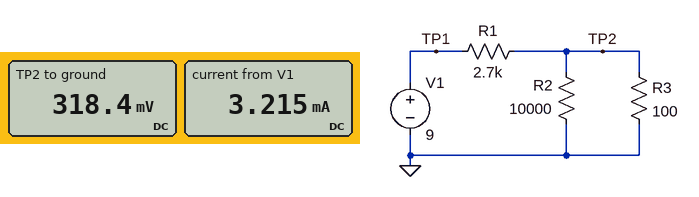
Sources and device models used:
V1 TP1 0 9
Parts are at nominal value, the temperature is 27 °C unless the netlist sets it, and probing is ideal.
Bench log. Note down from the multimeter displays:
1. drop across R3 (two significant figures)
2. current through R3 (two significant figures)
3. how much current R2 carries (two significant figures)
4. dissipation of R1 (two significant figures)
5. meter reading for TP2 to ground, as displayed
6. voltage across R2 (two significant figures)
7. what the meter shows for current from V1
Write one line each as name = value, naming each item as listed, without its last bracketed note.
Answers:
drop across R3 = 320 mV
current through R3 = 3.2 mA
how much current R2 carries = 32 µA
dissipation of R1 = 28 mW
meter reading for TP2 to ground, as displayed = 318.4 mV
voltage across R2 = 320 mV
what the meter shows for current from V1 = 3.215 mA
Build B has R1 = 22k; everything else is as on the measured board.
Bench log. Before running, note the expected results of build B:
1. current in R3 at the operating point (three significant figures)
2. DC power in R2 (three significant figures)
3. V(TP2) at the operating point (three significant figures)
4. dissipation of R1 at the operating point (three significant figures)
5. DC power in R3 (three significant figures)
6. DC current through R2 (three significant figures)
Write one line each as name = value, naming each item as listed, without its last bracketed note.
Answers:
current in R3 at the operating point = 403 µA
DC power in R2 = 163 nW
V(TP2) at the operating point = 40.3 mV
dissipation of R1 at the operating point = 3.65 mW
DC power in R3 = 16.3 µW
DC current through R2 = 4.03 µA
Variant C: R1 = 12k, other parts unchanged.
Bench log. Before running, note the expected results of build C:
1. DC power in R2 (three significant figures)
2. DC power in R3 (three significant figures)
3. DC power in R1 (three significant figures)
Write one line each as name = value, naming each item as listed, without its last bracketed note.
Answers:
DC power in R2 = 542 nW
DC power in R3 = 54.2 µW
DC power in R1 = 6.64 mW
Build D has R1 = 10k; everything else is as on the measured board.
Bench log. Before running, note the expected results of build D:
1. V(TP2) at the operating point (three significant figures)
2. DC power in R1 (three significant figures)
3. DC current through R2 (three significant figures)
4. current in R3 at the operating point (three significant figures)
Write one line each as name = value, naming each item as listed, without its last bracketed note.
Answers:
V(TP2) at the operating point = 88.2 mV
DC power in R1 = 7.94 mW
DC current through R2 = 8.82 µA
current in R3 at the operating point = 882 µA
